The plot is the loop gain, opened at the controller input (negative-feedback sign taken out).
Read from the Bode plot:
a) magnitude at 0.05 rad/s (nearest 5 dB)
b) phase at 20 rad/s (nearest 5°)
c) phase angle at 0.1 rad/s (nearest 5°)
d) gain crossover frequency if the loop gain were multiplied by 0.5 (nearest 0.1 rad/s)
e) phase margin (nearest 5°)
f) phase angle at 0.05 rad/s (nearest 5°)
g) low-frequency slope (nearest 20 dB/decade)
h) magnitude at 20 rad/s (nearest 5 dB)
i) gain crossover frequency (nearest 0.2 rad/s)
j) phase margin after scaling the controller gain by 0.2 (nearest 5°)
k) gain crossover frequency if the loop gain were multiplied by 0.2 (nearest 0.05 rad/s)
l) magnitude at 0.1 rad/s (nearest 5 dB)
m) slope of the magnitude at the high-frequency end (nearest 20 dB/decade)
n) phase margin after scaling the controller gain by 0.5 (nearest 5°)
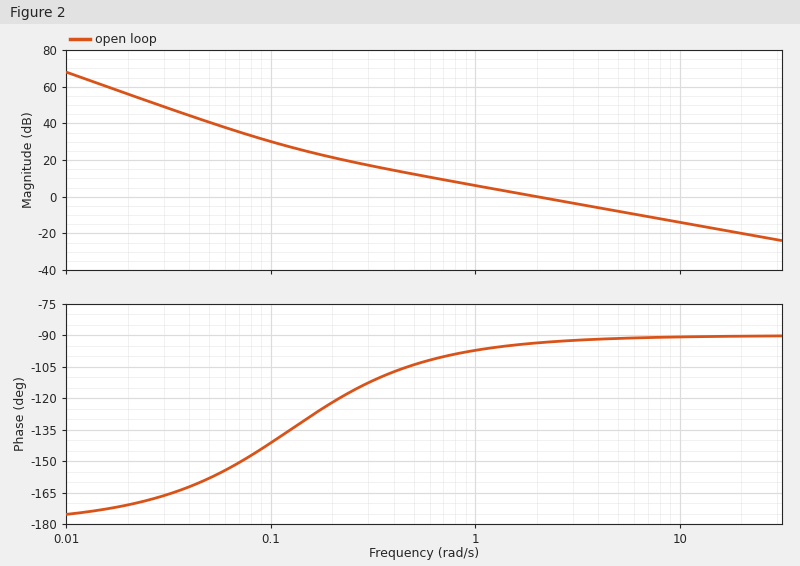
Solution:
40 dB
-90°
-140°
1.0 rad/s
85°
-160°
-40 dB/decade
-20 dB
2.0 rad/s
75°
0.40 rad/s
30 dB
-20 dB/decade
85°
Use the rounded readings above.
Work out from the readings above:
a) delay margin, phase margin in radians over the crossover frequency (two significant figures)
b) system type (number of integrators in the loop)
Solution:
0.74 s
2
